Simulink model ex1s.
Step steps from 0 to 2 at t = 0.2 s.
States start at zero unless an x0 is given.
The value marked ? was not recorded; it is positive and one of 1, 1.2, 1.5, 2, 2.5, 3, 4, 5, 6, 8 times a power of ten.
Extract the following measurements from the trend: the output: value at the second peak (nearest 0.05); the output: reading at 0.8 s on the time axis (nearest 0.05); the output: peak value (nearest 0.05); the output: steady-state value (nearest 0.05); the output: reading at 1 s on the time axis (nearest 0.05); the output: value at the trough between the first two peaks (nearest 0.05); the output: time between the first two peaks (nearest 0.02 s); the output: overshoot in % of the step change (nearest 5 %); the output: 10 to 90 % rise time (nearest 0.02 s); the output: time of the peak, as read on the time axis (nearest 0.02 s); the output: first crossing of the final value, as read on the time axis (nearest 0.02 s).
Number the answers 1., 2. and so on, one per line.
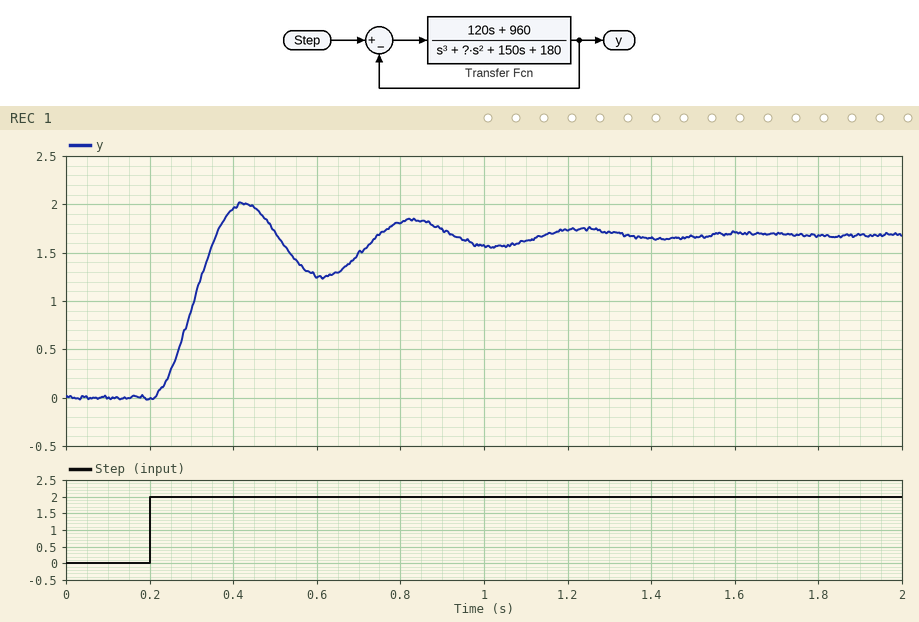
1. 1.85
2. 1.80
3. 2.00
4. 1.70
5. 1.55
6. 1.25
7. 0.40 s
8. 20 %
9. 0.10 s
10. 0.42 s
11. 0.36 s
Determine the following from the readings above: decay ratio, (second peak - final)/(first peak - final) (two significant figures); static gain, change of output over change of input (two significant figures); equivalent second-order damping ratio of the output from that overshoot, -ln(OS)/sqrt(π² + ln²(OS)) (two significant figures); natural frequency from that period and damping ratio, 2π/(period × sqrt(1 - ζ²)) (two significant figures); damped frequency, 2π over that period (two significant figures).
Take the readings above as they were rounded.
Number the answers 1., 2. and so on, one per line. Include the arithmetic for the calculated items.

1. (1.85 - 1.7) / (2 - 1.7) = 0.50
2. (1.7 - 0) / (2 - 0) = 0.85
3. ln(0.2) = -1.609; 1.609 / sqrt(9.870 + 2.590) = 0.46
4. 2π / (0.4 × sqrt(1 - 0.46²)) = 18 rad/s
5. 2π / 0.4 = 16 rad/s
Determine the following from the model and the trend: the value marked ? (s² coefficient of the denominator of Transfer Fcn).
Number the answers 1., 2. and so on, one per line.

1. 10
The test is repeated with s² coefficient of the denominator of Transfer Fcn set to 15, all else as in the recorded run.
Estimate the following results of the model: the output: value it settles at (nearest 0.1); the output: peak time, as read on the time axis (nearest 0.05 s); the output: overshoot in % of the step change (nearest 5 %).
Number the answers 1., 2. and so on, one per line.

1. 1.7
2. 0.45 s
3. 10 %
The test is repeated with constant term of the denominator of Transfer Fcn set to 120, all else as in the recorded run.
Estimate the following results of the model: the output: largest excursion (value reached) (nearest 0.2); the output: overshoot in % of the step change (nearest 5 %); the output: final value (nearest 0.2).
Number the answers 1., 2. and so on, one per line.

1. 2.0
2. 15 %
3. 1.8
